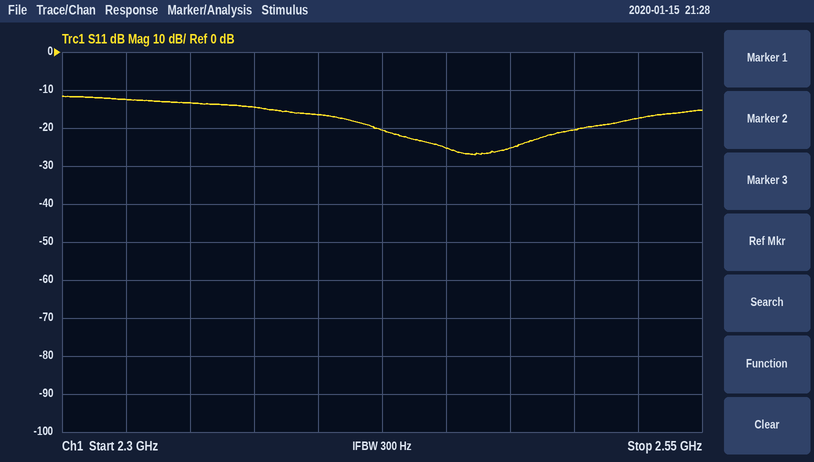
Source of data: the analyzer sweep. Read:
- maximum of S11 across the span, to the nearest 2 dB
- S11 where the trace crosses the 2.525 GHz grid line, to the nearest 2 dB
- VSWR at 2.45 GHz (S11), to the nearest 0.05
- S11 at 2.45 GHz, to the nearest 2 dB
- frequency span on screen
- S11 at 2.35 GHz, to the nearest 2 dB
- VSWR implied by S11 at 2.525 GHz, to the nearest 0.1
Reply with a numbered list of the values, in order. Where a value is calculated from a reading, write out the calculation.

1. -12 dB
2. -18 dB
3. |Γ| = 10^(-26/20) = 0.0501; VSWR = (1 + 0.0501)/(1 − 0.0501) ≈ 1.11, so 1.10 to the nearest 0.05
4. -26 dB
5. 250 MHz
6. -14 dB
7. |Γ| = 10^(-18/20) = 0.1259; VSWR = (1 + 0.1259)/(1 − 0.1259) ≈ 1.3
